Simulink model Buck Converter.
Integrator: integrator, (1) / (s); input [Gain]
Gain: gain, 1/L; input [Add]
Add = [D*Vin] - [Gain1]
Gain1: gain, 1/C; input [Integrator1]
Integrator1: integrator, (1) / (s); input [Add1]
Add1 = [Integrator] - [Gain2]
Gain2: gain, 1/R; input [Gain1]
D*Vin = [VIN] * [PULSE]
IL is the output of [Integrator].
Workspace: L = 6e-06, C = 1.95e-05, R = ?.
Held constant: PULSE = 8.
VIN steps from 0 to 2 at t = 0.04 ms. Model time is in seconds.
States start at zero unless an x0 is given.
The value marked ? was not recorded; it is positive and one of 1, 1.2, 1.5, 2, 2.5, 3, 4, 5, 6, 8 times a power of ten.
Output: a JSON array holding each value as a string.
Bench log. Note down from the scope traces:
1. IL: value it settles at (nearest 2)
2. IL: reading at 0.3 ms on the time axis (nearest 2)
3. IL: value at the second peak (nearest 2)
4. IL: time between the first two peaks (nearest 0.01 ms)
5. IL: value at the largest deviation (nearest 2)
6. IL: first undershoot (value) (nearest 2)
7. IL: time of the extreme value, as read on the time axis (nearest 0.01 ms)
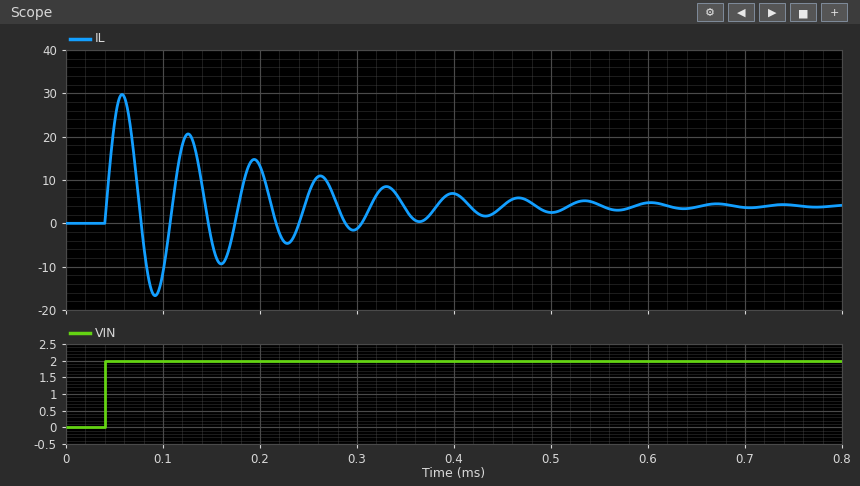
["4", "-2", "20", "0.07 ms", "30", "-16", "0.06 ms"]
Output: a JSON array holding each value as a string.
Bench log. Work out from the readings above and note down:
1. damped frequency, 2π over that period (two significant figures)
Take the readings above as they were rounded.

["90 rad/ms"]
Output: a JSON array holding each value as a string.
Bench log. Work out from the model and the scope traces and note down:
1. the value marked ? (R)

["4"]
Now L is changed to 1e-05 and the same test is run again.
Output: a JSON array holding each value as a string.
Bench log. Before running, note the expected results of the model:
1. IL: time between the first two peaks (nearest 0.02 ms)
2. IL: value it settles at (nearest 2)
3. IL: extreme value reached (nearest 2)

["0.08 ms", "4", "24"]
